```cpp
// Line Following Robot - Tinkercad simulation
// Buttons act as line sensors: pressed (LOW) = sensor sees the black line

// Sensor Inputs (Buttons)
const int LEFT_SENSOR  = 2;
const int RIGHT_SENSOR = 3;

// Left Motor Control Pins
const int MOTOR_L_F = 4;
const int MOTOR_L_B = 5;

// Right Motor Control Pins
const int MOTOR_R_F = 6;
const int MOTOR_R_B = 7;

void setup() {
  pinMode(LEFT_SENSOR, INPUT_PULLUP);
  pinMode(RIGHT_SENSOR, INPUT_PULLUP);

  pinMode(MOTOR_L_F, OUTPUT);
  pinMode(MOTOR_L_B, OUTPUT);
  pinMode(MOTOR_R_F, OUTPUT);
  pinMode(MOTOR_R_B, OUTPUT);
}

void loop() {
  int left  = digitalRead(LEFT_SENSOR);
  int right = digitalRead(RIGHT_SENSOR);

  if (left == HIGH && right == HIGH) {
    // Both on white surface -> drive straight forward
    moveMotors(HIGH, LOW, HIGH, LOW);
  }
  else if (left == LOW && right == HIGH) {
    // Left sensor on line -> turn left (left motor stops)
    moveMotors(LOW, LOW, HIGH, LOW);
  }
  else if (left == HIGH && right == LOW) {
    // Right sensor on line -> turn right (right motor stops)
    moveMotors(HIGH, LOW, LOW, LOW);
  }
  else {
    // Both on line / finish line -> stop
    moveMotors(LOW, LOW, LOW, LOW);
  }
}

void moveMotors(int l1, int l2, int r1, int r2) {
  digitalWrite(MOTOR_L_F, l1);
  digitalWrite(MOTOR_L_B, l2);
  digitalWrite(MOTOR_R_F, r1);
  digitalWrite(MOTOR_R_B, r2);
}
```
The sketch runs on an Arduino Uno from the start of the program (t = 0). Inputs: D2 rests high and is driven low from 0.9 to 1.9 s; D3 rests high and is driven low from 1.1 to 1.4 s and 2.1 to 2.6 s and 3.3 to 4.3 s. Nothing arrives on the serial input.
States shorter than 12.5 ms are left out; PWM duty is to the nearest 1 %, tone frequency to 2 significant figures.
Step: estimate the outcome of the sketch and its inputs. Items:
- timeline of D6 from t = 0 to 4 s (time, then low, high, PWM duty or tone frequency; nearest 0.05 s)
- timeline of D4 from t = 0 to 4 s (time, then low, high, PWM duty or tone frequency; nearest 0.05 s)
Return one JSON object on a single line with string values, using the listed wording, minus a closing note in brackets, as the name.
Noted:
{"timeline of D6 from t = 0 to 4 s": "0 s high; 1.1 s low; 1.4 s high; 2.1 s low; 2.6 s high; 3.3 s low", "timeline of D4 from t = 0 to 4 s": "0 s high; 0.9 s low; 1.9 s high"}
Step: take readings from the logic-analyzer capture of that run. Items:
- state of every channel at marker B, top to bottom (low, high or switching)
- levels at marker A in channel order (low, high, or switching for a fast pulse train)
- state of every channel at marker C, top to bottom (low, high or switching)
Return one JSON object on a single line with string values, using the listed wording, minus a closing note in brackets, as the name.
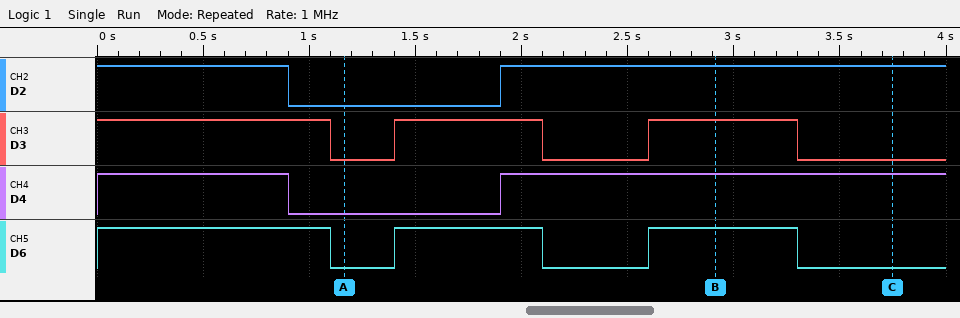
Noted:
{"state of every channel at marker B, top to bottom": "D2 high, D3 high, D4 high, D6 high", "levels at marker A in channel order": "D2 low, D3 low, D4 low, D6 low", "state of every channel at marker C, top to bottom": "D2 high, D3 low, D4 high, D6 low"}
